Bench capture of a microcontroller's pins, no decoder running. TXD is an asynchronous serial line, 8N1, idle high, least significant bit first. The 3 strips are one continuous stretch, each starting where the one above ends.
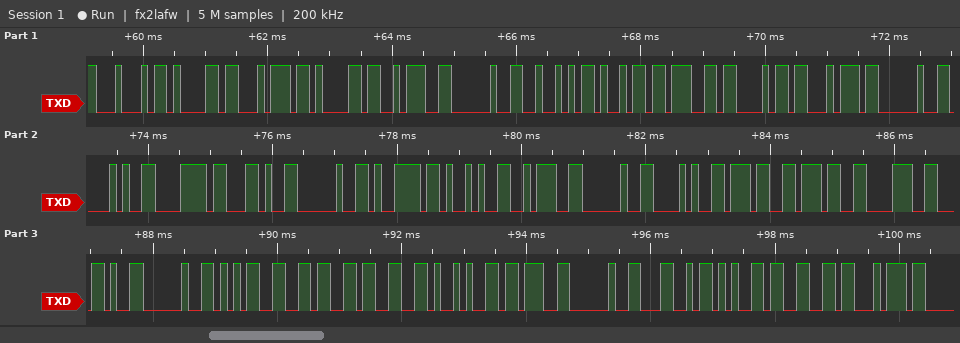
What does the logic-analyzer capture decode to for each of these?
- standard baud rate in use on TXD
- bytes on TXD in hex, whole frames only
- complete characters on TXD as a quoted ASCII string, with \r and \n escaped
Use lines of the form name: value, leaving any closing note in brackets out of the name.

standard baud rate in use on TXD: 9600 baud
bytes on TXD in hex, whole frames only: 44 61 74 61 3A 20 52 69 67 68 74 20 28 78 2C 20 79 29 3A 20 28 37 37 38 2C 20 35 36 33 29 3B 20 4C 65 66 74
complete characters on TXD as a quoted ASCII string, with \r and \n escaped: "Data: Right (x, y): (778, 563); Left"
